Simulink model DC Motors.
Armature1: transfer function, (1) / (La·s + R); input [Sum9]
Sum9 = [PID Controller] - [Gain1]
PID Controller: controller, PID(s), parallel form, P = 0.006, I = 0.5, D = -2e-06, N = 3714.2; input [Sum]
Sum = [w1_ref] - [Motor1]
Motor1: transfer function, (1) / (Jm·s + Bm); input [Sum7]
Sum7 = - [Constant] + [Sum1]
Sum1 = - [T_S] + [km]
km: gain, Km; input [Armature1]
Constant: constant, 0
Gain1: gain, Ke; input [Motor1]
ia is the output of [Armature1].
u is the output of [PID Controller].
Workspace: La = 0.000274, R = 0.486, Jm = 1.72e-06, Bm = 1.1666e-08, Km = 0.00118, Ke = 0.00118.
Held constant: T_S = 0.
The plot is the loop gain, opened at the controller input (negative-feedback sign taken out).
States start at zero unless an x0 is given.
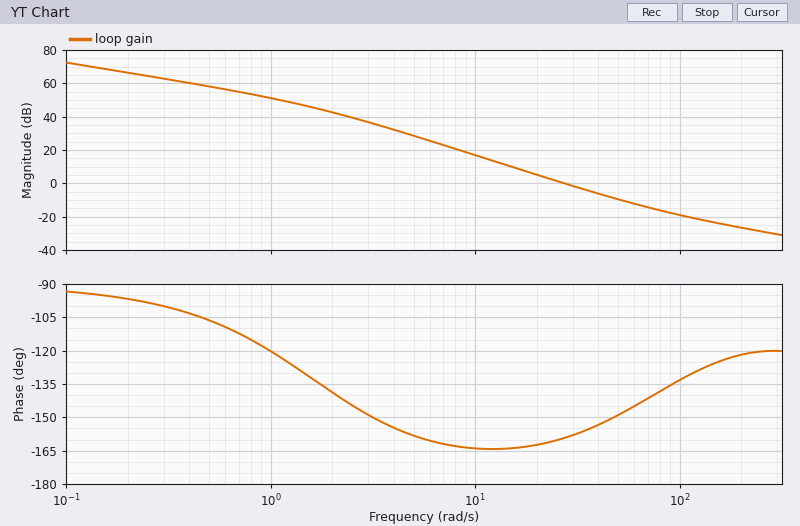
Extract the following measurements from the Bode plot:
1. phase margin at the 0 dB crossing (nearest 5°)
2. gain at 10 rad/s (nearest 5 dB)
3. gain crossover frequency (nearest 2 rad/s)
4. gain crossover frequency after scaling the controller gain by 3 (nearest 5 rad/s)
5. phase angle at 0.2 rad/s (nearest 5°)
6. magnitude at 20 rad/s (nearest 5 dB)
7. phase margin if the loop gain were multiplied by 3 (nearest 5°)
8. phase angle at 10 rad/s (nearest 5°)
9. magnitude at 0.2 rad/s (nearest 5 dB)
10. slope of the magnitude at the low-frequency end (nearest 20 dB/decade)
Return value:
20°
15 dB
28 rad/s
50 rad/s
-95°
5 dB
30°
-165°
65 dB
-20 dB/decade
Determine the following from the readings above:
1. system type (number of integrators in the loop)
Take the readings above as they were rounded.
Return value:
1
